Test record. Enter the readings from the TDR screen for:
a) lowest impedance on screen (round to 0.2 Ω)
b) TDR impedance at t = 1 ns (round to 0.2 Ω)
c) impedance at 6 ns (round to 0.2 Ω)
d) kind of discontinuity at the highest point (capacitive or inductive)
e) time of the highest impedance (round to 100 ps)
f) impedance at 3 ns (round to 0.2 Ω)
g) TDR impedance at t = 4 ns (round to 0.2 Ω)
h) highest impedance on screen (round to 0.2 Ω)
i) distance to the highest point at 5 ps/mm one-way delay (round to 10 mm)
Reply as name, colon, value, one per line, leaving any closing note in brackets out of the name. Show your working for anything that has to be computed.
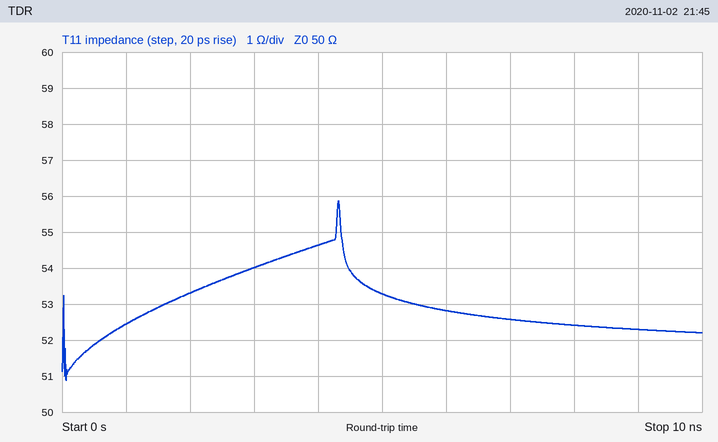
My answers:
lowest impedance on screen: 50.8 Ω
TDR impedance at t = 1 ns: 52.4 Ω
impedance at 6 ns: 52.8 Ω
kind of discontinuity at the highest point: inductive
time of the highest impedance: 4.3 ns
impedance at 3 ns: 54.0 Ω
TDR impedance at t = 4 ns: 54.6 Ω
highest impedance on screen: 55.8 Ω
distance to the highest point at 5 ps/mm one-way delay: 4.3 ns / 2 / 5 ps/mm ≈ 430 mm
